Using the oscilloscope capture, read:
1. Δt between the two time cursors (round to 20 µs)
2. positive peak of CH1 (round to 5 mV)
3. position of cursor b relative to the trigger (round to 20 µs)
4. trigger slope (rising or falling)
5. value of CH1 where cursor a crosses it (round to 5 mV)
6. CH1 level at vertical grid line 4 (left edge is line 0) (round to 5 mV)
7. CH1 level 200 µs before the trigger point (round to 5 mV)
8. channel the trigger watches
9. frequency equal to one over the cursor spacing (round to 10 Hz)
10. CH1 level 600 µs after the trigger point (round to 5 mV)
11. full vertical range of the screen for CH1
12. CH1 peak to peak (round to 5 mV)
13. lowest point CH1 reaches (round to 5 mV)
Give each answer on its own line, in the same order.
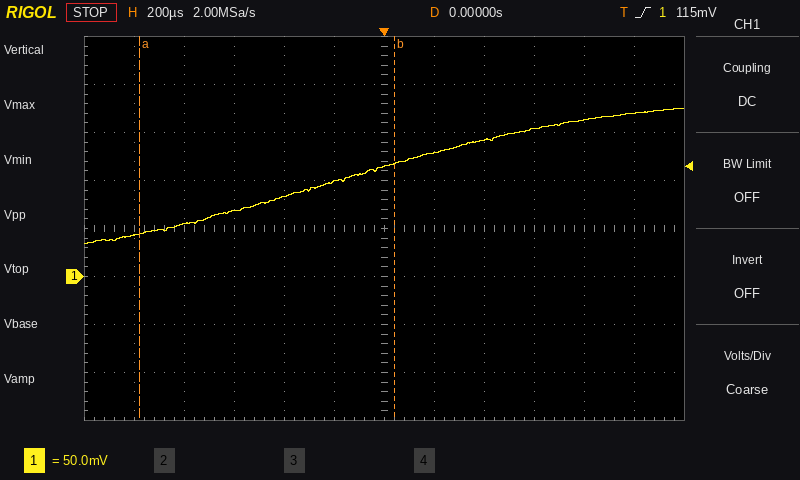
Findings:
1.02 ms
175 mV
+40 µs
rising
45 mV
85 mV
100 mV
CH1
980 Hz
155 mV
400 mV
140 mV
35 mV
